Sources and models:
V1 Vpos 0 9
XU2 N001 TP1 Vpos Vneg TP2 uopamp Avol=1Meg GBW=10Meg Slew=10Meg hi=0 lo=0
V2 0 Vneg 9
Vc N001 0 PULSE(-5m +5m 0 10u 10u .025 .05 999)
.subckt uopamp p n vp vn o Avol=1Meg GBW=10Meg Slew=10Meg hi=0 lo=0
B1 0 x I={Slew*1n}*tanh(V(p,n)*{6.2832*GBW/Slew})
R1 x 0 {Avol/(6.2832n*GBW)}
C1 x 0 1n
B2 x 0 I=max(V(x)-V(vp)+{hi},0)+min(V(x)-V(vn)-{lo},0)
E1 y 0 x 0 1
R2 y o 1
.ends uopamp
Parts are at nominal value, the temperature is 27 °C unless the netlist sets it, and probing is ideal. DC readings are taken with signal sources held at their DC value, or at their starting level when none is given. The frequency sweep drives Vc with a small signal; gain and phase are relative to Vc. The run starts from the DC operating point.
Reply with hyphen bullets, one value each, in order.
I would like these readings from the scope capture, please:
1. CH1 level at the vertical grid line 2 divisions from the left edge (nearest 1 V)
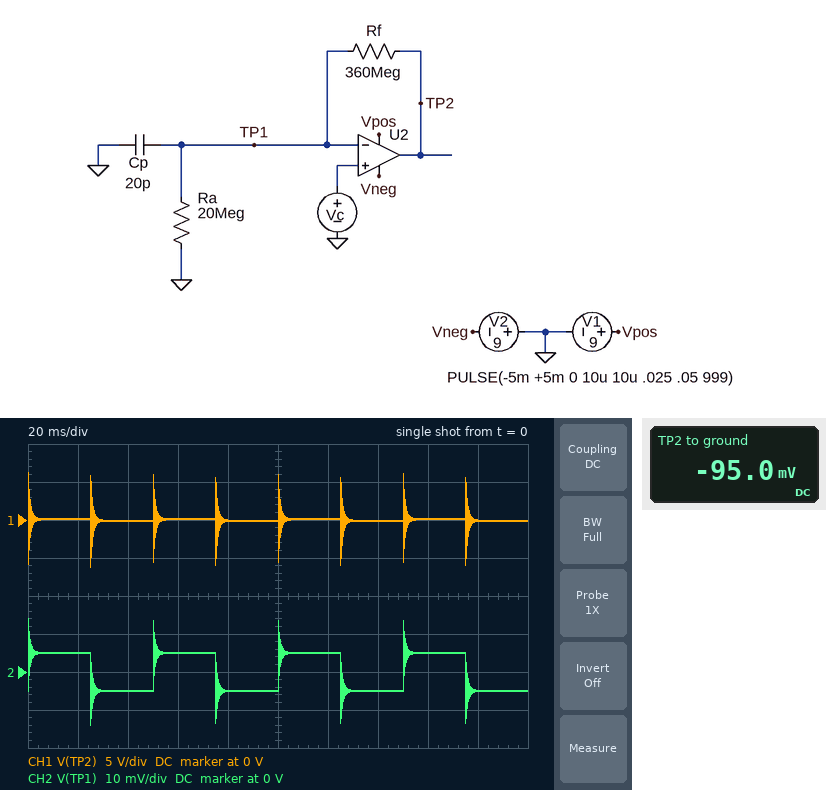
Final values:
- 0 V
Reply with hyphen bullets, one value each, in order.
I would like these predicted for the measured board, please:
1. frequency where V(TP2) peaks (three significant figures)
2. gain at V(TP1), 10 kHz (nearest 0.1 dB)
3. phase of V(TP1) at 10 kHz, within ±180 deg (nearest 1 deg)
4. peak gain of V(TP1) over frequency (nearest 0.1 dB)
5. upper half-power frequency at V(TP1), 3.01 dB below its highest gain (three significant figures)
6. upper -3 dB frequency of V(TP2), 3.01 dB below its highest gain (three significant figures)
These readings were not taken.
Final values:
- 14.9 kHz
- 5.2 dB
- -2 deg
- 30.8 dB
- 15.1 kHz
- 15.1 kHz
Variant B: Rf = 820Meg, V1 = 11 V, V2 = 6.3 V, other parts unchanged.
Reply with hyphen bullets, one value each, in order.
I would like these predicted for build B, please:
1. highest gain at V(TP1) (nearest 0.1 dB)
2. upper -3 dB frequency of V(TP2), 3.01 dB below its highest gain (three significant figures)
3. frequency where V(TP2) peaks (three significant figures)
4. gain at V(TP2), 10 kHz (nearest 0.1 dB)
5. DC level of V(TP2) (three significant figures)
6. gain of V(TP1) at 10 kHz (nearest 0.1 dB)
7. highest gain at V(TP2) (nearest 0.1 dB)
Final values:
- 27.5 dB
- 10.1 kHz
- 9.85 kHz
- 85.8 dB
- -210 mV
- 25.6 dB
- 87.6 dB
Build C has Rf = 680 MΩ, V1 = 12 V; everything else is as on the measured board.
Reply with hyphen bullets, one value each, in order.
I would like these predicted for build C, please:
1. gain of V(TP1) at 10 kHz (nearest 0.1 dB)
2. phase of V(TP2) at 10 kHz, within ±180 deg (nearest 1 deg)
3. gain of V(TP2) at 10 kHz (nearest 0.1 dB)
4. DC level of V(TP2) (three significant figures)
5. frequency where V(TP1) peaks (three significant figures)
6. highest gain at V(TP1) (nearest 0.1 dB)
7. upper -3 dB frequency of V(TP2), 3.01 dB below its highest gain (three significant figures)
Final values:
- 16.5 dB
- 74 deg
- 75.1 dB
- -175 mV
- 10.8 kHz
- 28.2 dB
- 11.0 kHz
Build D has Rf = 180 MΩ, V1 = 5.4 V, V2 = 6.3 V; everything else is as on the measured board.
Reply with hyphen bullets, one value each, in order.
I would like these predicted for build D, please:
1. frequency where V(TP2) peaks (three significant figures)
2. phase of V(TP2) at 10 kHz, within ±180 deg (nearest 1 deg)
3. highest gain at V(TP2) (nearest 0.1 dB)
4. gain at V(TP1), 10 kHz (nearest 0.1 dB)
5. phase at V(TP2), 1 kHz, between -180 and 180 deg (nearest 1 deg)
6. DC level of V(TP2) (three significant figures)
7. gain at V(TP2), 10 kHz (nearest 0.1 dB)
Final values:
- 21.0 kHz
- 87 deg
- 86.9 dB
- 2.2 dB
- 66 deg
- -50.0 mV
- 49.3 dB
